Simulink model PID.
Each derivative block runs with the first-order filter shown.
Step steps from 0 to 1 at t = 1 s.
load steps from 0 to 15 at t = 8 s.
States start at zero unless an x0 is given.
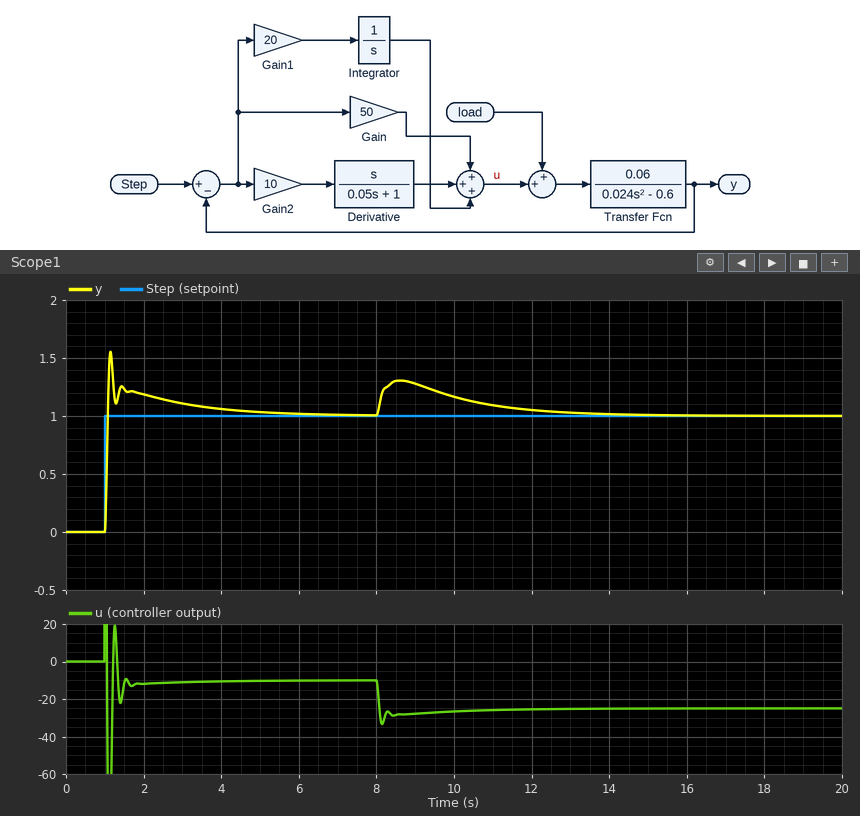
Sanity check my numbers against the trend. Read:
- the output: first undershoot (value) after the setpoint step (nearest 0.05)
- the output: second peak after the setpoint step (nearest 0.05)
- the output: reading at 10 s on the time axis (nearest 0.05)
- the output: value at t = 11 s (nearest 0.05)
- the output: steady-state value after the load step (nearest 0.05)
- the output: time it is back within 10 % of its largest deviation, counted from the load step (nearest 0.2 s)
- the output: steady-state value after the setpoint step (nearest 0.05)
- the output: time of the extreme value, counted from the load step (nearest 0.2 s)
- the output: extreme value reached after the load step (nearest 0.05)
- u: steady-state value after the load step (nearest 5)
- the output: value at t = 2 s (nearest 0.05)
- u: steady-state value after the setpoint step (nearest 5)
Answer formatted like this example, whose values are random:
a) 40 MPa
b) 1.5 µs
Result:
a) 1.10
b) 1.25
c) 1.15
d) 1.10
e) 1.00
f) 5.0 s
g) 1.00
h) 0.6 s
i) 1.30
j) -25
k) 1.20
l) -10
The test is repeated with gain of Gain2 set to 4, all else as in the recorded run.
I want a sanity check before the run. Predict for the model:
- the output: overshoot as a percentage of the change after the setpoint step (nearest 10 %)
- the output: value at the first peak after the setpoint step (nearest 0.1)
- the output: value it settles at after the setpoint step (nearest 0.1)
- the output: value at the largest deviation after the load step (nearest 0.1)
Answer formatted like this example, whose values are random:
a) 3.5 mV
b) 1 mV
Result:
a) 80 %
b) 1.8
c) 1.0
d) 1.4
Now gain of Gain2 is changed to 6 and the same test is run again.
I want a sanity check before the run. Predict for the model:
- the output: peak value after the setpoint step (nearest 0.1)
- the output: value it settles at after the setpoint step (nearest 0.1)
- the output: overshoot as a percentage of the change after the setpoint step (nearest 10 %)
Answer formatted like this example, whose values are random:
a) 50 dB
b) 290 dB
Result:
a) 1.7
b) 1.0
c) 70 %
